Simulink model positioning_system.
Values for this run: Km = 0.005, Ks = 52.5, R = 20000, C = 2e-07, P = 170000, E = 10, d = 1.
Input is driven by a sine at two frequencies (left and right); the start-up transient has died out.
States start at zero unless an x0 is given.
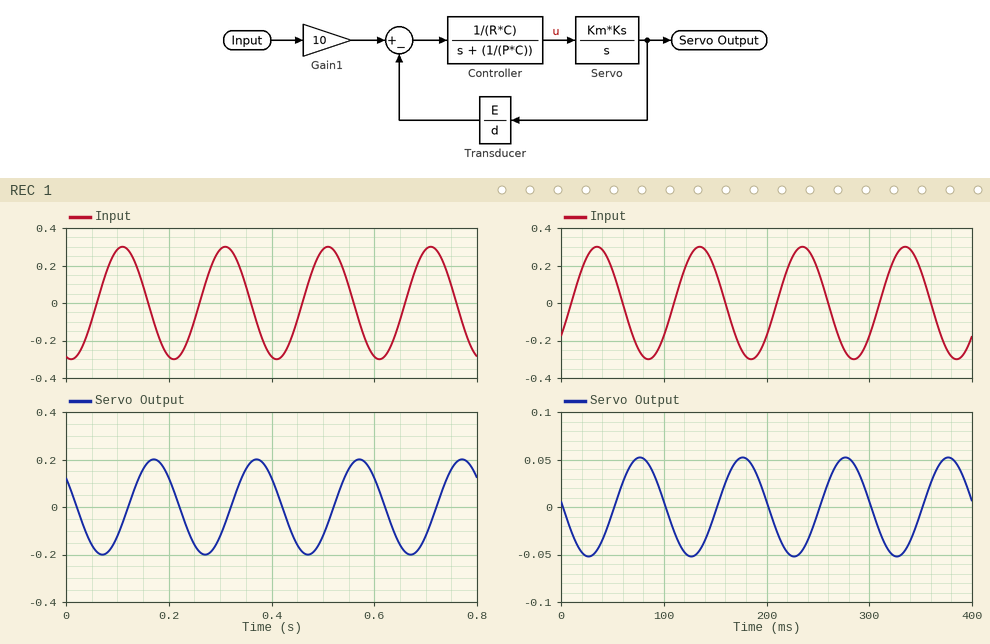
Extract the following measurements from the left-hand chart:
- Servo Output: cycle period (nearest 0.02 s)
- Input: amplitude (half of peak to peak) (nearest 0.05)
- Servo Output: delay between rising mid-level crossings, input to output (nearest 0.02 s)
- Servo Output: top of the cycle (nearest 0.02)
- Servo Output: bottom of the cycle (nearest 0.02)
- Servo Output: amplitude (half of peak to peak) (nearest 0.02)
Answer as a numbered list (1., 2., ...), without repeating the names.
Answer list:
1. 0.20 s
2. 0.30
3. 0.06 s
4. 0.20
5. -0.20
6. 0.20
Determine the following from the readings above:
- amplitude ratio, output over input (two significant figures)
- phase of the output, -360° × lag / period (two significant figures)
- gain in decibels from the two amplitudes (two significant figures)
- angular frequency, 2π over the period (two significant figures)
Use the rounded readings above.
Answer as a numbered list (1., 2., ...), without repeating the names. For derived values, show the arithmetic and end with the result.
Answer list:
1. 0.2 / 0.3 = 0.67
2. -360 × 0.06 / 0.2 = -110°
3. 20 log10(0.2 / 0.3) = -3.5 dB
4. 2π / 0.2 = 31 rad/s
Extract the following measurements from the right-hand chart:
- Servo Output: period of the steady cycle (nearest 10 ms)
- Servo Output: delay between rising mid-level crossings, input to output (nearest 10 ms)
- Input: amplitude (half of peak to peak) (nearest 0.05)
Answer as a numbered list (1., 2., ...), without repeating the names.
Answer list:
1. 100 ms
2. 40 ms
3. 0.30
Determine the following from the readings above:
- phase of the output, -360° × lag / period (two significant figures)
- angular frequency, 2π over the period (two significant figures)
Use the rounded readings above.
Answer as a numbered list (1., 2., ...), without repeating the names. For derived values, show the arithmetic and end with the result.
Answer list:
1. -360 × 40 / 100 = -140°
2. 2π / 100 = 0.063 rad/ms
